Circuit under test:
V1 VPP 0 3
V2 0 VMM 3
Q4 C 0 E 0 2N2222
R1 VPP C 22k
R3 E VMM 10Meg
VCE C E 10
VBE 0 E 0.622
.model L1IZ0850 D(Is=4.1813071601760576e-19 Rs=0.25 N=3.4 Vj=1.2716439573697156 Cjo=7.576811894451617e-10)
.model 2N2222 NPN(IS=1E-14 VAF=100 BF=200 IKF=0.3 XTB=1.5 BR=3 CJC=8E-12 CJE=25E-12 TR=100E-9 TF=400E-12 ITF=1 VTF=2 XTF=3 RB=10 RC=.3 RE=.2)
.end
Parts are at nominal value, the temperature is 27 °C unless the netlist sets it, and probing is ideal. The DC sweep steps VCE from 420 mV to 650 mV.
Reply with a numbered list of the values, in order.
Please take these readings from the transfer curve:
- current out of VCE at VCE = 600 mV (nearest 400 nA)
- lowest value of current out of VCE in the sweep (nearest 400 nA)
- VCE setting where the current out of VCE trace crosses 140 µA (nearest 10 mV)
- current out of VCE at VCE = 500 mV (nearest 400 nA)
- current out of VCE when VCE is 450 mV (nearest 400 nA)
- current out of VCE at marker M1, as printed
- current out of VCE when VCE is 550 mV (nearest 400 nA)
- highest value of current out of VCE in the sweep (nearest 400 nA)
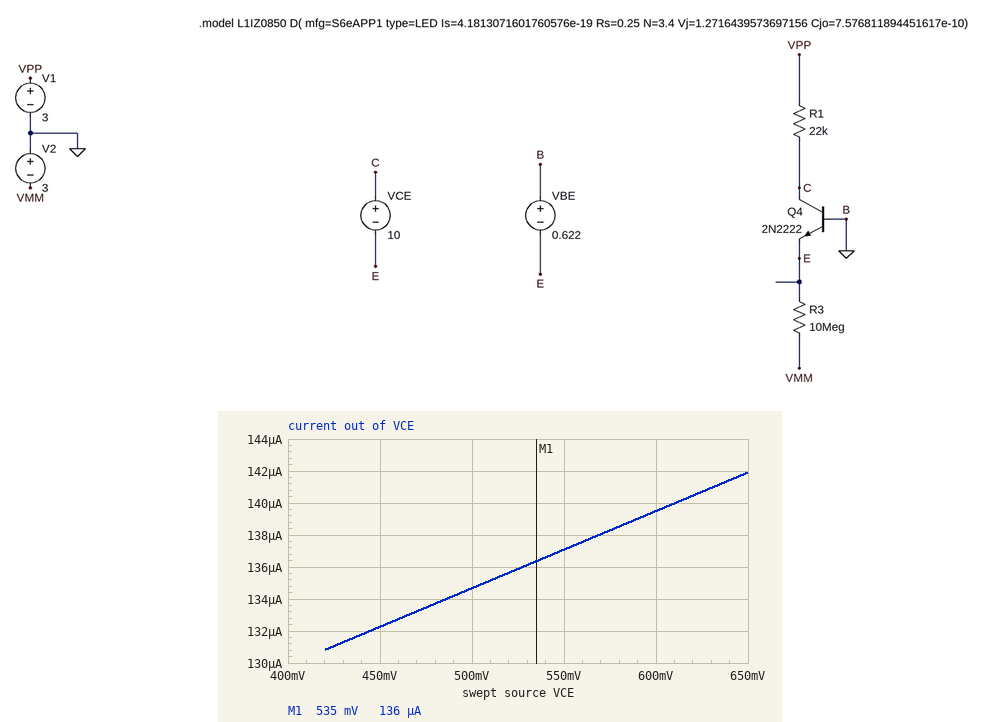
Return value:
1. 139.6 µA
2. 130.8 µA
3. 610 mV
4. 134.8 µA
5. 132.4 µA
6. 136 µA
7. 137.2 µA
8. 142.0 µA
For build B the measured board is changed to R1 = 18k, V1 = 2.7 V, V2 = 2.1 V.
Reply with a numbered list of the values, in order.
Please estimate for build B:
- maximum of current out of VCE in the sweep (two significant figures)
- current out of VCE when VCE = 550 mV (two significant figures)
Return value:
1. 130 µA
2. 120 µA
